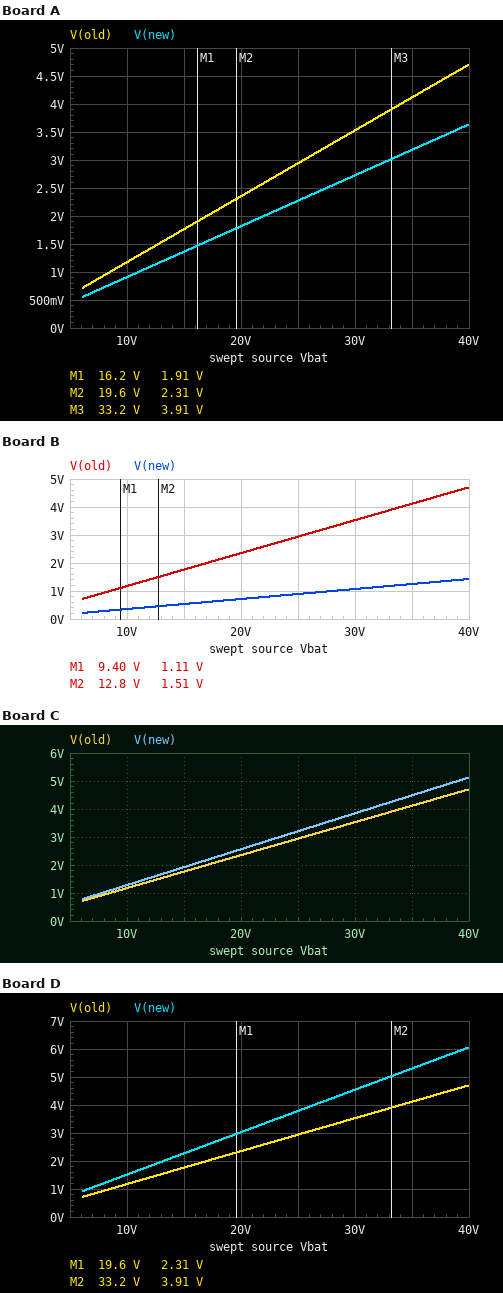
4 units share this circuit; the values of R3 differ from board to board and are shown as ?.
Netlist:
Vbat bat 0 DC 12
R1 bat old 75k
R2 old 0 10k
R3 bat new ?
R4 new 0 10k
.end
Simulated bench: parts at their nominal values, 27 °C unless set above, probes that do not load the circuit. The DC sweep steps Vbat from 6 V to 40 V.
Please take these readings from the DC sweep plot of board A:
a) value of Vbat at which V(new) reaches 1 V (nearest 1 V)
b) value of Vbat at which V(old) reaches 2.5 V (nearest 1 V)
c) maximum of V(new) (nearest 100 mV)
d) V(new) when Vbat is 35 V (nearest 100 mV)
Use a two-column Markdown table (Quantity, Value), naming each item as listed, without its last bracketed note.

| Quantity | Value |
|---|---|
| value of Vbat at which V(new) reaches 1 V | 11 V |
| value of Vbat at which V(old) reaches 2.5 V | 21 V |
| maximum of V(new) | 3.6 V |
| V(new) when Vbat is 35 V | 3.2 V |
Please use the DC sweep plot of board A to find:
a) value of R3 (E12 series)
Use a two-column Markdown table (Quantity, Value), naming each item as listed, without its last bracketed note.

| Quantity | Value |
|---|---|
| value of R3 | 100 kΩ |
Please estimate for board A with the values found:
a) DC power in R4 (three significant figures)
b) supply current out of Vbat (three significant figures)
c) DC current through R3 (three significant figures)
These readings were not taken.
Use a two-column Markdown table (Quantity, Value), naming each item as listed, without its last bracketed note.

| Quantity | Value |
|---|---|
| DC power in R4 | 119 µW |
| supply current out of Vbat | 250 µA |
| DC current through R3 | 109 µA |
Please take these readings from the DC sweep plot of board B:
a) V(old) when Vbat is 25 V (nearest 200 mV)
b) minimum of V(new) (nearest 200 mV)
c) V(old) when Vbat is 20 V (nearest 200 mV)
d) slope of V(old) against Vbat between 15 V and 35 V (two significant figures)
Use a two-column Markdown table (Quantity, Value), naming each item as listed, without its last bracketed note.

| Quantity | Value |
|---|---|
| V(old) when Vbat is 25 V | 3.0 V |
| minimum of V(new) | 200 mV |
| V(old) when Vbat is 20 V | 2.4 V |
| slope of V(old) against Vbat between 15 V and 35 V | 0.12 V/V |
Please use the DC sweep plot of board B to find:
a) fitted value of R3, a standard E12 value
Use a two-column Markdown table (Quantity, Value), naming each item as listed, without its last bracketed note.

| Quantity | Value |
|---|---|
| fitted value of R3, a standard E12 value | 270 kΩ |
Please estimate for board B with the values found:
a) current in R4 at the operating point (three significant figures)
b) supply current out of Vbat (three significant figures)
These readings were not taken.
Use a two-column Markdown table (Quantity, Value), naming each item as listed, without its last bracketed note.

| Quantity | Value |
|---|---|
| current in R4 at the operating point | 42.9 µA |
| supply current out of Vbat | 184 µA |
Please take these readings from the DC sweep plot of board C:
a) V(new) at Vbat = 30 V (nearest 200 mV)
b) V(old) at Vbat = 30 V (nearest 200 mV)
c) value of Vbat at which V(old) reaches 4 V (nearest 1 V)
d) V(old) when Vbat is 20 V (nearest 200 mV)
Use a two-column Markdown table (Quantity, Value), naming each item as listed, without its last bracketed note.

| Quantity | Value |
|---|---|
| V(new) at Vbat = 30 V | 3.8 V |
| V(old) at Vbat = 30 V | 3.6 V |
| value of Vbat at which V(old) reaches 4 V | 34 V |
| V(old) when Vbat is 20 V | 2.4 V |
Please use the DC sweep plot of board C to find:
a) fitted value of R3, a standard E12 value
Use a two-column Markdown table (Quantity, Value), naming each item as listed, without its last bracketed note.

| Quantity | Value |
|---|---|
| fitted value of R3, a standard E12 value | 68 kΩ |
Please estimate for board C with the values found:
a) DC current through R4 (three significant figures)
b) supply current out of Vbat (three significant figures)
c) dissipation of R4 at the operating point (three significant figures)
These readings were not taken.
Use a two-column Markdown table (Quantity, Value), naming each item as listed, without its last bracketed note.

| Quantity | Value |
|---|---|
| DC current through R4 | 154 µA |
| supply current out of Vbat | 295 µA |
| dissipation of R4 at the operating point | 237 µW |
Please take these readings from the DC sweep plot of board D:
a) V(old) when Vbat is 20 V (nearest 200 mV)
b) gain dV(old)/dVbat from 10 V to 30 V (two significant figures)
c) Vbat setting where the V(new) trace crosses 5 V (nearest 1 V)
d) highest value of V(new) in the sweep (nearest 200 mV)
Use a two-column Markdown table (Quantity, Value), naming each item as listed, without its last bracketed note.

| Quantity | Value |
|---|---|
| V(old) when Vbat is 20 V | 2.4 V |
| gain dV(old)/dVbat from 10 V to 30 V | 0.12 V/V |
| Vbat setting where the V(new) trace crosses 5 V | 33 V |
| highest value of V(new) in the sweep | 6.0 V |
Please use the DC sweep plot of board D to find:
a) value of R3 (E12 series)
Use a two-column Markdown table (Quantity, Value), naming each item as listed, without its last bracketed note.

| Quantity | Value |
|---|---|
| value of R3 | 56 kΩ |
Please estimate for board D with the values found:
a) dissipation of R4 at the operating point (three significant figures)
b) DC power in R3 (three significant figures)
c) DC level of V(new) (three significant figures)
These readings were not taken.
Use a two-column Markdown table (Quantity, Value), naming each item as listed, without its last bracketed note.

| Quantity | Value |
|---|---|
| dissipation of R4 at the operating point | 331 µW |
| DC power in R3 | 1.85 mW |
| DC level of V(new) | 1.82 V |
